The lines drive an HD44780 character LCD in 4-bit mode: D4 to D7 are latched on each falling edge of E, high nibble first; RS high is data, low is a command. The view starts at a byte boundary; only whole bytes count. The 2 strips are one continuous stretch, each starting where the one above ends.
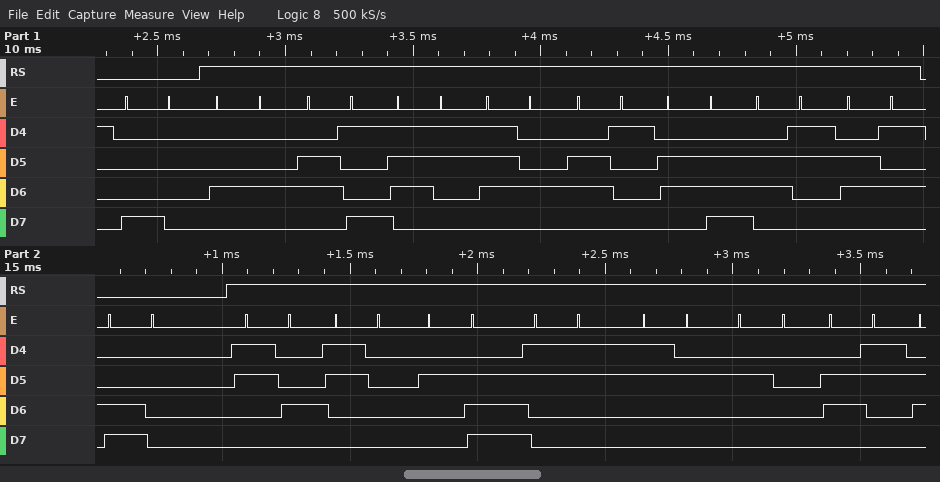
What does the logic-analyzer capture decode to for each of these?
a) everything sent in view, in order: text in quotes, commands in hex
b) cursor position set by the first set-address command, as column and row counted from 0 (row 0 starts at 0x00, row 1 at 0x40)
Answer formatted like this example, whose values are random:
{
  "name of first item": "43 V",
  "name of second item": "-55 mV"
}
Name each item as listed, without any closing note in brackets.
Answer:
{
  "everything sent in view, in order: text in quotes, commands in hex": "0x80 \"Distance\" 0xC0 \"40.32 c\"",
  "cursor position set by the first set-address command, as column and row counted from 0": "column 0, row 0"
}
